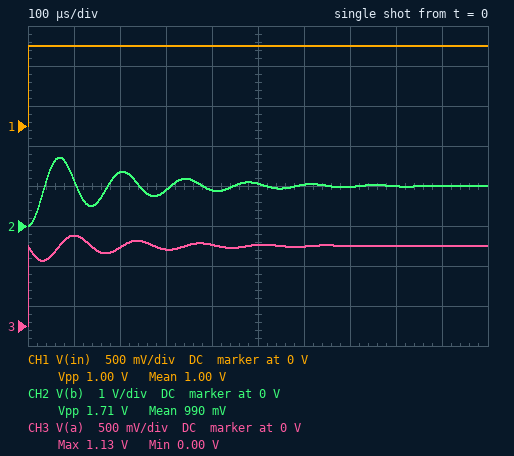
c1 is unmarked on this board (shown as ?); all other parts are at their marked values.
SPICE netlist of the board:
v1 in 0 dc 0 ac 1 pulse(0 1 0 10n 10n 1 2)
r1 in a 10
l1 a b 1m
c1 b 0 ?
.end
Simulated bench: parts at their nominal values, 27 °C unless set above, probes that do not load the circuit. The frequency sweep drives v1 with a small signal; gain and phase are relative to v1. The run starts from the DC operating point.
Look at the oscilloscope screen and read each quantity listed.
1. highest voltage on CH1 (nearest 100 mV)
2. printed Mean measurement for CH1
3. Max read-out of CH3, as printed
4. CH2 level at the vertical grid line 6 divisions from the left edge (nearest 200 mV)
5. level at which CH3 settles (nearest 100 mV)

1.0 V
1.00 V
1.13 V
1.0 V
1.0 V
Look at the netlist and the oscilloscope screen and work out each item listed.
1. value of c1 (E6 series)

470 nF
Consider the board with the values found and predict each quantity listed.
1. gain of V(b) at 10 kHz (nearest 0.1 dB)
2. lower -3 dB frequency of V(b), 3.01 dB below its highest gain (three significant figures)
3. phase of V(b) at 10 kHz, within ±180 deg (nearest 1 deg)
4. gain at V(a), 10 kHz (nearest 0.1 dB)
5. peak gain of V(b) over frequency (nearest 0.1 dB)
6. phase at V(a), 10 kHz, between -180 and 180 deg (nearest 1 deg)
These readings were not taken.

0.9 dB
6.40 kHz
-161 deg
-0.5 dB
13.3 dB
19 deg
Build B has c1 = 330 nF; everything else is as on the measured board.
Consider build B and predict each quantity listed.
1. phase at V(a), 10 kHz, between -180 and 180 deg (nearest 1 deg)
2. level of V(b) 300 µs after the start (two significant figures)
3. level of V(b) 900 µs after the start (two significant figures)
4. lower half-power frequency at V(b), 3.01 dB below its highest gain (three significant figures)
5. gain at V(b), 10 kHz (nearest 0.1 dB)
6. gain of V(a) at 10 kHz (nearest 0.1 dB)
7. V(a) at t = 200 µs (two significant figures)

34 deg
1.2 V
990 mV
7.85 kHz
8.7 dB
-1.7 dB
1.1 V
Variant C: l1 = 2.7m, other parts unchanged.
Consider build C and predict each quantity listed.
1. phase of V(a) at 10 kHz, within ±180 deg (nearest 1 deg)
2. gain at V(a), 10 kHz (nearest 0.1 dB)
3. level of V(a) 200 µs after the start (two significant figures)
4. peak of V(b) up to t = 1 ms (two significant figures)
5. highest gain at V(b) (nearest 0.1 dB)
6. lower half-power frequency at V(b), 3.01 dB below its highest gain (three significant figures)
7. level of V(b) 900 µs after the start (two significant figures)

4 deg
0 dB
1.1 V
1.8 V
17.6 dB
4.14 kHz
810 mV
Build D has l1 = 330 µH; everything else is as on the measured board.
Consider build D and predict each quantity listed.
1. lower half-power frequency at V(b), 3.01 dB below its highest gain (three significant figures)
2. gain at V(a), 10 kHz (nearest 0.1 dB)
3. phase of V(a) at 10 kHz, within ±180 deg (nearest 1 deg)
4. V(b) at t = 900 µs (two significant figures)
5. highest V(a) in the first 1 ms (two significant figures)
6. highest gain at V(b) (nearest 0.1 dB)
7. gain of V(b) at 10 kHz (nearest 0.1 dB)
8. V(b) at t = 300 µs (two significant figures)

9.55 kHz
-2.0 dB
-37 deg
1.0 V
1.2 V
8.6 dB
6.2 dB
1.0 V
